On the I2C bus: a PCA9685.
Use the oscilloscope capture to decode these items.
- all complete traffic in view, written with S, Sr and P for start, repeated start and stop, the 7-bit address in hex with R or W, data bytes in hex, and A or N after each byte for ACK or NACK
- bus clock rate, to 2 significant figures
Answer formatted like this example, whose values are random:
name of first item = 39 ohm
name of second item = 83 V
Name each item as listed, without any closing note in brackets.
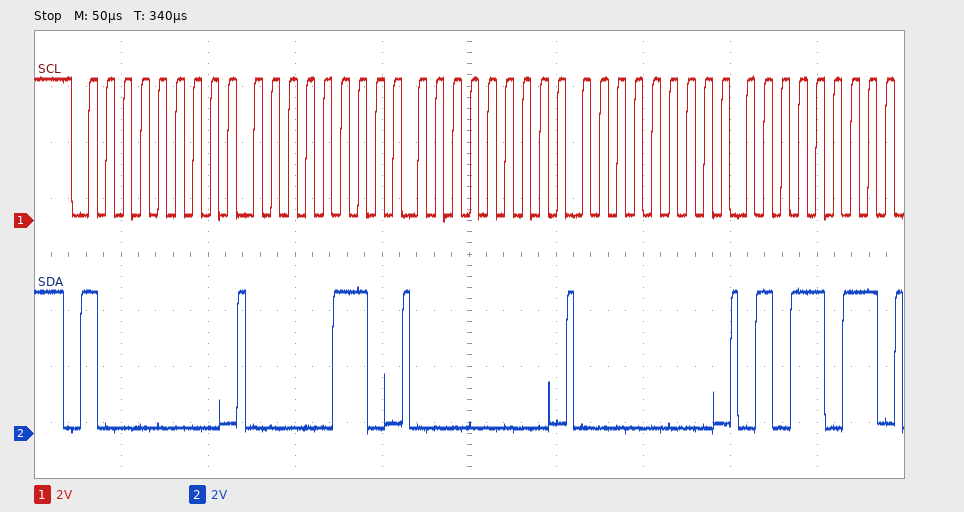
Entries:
all complete traffic in view, written with S, Sr and P for start, repeated start and stop, the 7-bit address in hex with R or W, data bytes in hex, and A or N after each byte for ACK or NACK = S 40W A 06 A 00 A 00 A 5B A
bus clock rate, to 2 significant figures = 100 kHz
